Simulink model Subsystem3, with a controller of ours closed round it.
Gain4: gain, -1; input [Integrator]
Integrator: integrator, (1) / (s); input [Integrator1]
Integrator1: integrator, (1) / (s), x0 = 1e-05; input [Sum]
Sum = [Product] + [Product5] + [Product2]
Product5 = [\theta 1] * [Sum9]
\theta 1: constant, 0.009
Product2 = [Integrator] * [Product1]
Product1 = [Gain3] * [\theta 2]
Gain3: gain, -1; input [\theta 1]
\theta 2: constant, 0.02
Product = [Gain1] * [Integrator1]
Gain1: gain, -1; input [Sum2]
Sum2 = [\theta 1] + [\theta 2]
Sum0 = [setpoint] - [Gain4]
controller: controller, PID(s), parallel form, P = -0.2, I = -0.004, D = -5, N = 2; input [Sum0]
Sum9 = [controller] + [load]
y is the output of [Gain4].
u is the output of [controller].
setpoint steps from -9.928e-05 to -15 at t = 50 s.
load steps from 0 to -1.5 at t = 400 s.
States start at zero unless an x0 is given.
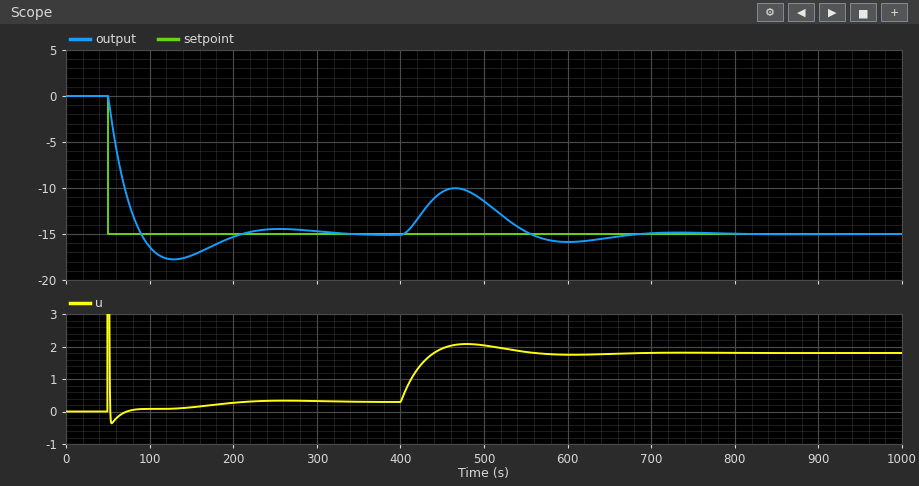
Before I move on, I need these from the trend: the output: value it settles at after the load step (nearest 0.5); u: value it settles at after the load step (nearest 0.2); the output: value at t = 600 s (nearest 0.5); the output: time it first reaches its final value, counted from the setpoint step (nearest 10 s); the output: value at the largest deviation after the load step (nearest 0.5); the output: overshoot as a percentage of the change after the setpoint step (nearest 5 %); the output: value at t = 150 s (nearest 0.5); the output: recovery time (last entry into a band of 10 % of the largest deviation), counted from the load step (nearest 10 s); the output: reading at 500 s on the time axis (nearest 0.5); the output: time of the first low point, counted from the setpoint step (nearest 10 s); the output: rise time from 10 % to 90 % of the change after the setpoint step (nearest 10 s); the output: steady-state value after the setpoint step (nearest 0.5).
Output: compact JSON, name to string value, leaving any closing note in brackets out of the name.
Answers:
{"the output: value it settles at after the load step": "-15.0", "u: value it settles at after the load step": "1.8", "the output: value at t = 600 s": "-16.0", "the output: time it first reaches its final value, counted from the setpoint step": "40 s", "the output: value at the largest deviation after the load step": "-10.0", "the output: overshoot as a percentage of the change after the setpoint step": "20 %", "the output: value at t = 150 s": "-17.5", "the output: recovery time (last entry into a band of 10 % of the largest deviation), counted from the load step": "240 s", "the output: reading at 500 s on the time axis": "-11.5", "the output: time of the first low point, counted from the setpoint step": "80 s", "the output: rise time from 10 % to 90 % of the change after the setpoint step": "30 s", "the output: steady-state value after the setpoint step": "-15.0"}
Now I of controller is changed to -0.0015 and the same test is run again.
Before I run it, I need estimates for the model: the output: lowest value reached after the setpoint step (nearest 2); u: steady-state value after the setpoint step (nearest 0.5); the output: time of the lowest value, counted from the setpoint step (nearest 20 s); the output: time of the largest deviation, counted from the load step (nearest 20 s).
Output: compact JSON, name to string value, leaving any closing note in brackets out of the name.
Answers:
{"the output: lowest value reached after the setpoint step": "-16", "u: steady-state value after the setpoint step": "0.5", "the output: time of the lowest value, counted from the setpoint step": "80 s", "the output: time of the largest deviation, counted from the load step": "80 s"}
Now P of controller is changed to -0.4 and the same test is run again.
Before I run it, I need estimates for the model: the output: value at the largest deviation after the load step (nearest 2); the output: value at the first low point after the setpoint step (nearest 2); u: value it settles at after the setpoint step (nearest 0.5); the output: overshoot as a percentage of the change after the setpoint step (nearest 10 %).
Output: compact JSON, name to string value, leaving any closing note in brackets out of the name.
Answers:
{"the output: value at the largest deviation after the load step": "-12", "the output: value at the first low point after the setpoint step": "-18", "u: value it settles at after the setpoint step": "0.5", "the output: overshoot as a percentage of the change after the setpoint step": "20 %"}
